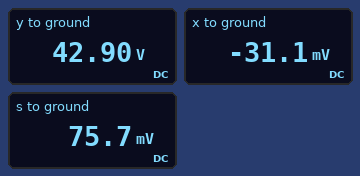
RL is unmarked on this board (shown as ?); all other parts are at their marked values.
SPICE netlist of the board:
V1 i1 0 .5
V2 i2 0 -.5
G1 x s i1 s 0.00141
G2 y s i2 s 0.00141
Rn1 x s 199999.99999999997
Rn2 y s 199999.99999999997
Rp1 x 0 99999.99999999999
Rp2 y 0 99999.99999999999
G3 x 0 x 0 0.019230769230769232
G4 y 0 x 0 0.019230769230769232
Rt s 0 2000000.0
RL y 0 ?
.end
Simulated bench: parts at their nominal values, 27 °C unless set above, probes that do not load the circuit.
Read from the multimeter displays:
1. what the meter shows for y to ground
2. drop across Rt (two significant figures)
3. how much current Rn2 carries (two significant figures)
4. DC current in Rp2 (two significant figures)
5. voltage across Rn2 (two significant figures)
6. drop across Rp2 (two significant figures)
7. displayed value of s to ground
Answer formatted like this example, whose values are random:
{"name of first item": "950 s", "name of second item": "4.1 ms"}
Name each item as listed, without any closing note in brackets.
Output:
{"what the meter shows for y to ground": "42.90 V", "drop across Rt": "76 mV", "how much current Rn2 carries": "210 µA", "DC current in Rp2": "430 µA", "voltage across Rn2": "43 V", "drop across Rp2": "43 V", "displayed value of s to ground": "75.7 mV"}
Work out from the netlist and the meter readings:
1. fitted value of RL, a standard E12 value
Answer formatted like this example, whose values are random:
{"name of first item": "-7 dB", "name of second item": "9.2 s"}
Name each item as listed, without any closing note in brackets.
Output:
{"fitted value of RL, a standard E12 value": "56 kΩ"}
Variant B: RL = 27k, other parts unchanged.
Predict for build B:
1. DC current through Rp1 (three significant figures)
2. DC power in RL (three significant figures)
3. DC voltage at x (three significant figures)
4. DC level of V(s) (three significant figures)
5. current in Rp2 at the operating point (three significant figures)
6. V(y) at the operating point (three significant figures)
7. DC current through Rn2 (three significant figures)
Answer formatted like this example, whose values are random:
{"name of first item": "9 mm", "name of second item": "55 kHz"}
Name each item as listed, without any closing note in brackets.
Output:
{"DC current through Rp1": "331 nA", "DC power in RL": "27.2 mW", "DC voltage at x": "-33.1 mV", "DC level of V(s)": "47.8 mV", "current in Rp2 at the operating point": "271 µA", "V(y) at the operating point": "27.1 V", "DC current through Rn2": "135 µA"}
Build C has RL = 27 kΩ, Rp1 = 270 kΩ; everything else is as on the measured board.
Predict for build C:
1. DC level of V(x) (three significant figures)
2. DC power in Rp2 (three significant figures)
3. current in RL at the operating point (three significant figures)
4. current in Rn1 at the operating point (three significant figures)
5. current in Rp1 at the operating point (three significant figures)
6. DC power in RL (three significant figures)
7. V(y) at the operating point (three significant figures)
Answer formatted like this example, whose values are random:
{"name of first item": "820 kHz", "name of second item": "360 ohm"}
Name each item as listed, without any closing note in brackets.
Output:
{"DC level of V(x)": "-33.1 mV", "DC power in Rp2": "7.34 mW", "current in RL at the operating point": "1.00 mA", "current in Rn1 at the operating point": "405 nA", "current in Rp1 at the operating point": "123 nA", "DC power in RL": "27.2 mW", "V(y) at the operating point": "27.1 V"}
